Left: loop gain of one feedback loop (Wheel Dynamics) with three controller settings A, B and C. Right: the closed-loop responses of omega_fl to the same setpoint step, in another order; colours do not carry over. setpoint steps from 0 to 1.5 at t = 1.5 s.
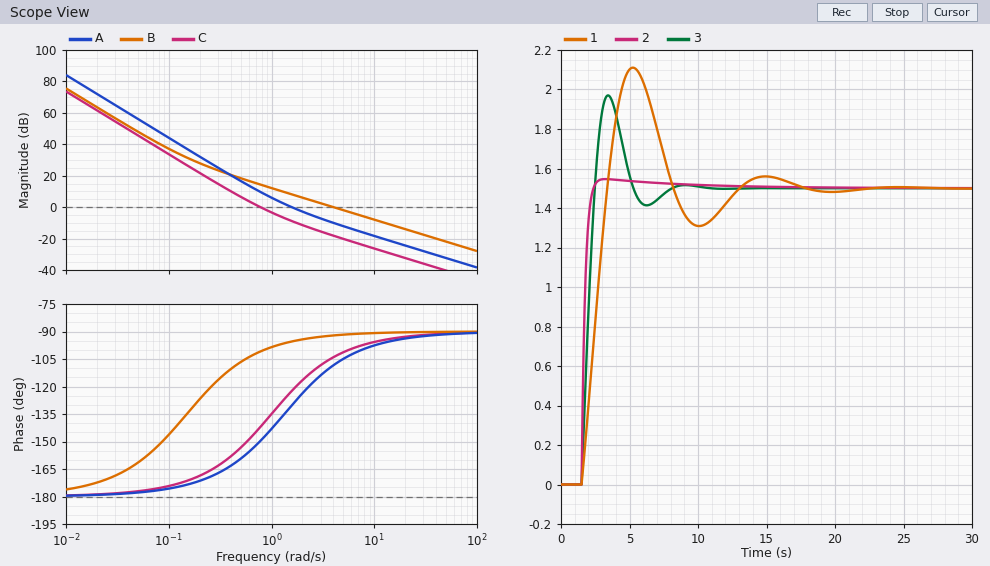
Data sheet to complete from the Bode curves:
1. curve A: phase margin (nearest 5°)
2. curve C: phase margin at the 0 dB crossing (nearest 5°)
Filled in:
50°
40°
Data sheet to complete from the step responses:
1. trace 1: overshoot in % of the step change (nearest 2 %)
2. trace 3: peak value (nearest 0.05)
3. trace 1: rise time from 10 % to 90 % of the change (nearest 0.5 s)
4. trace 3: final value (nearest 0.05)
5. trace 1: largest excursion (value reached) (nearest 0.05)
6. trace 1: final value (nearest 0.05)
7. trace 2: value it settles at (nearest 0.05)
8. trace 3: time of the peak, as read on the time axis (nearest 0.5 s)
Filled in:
40 %
1.95
1.5 s
1.50
2.10
1.50
1.50
3.5 s
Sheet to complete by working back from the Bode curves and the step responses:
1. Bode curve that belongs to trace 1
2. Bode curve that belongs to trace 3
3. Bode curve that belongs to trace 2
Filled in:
C
A
B
